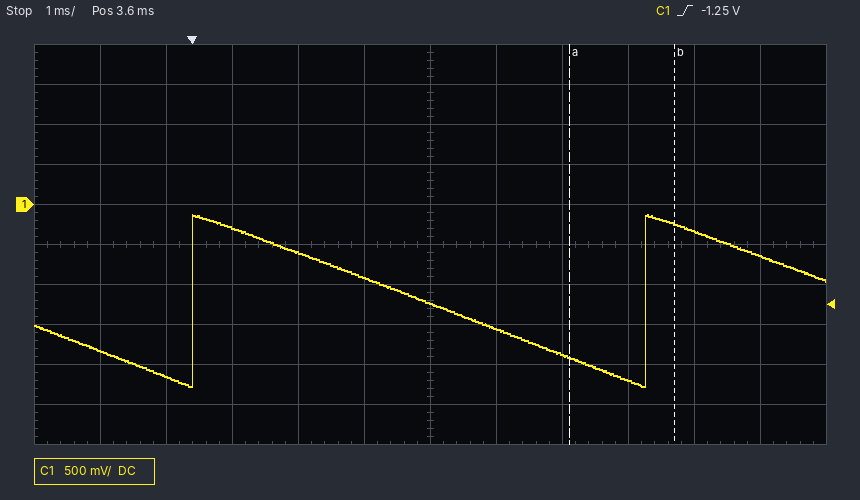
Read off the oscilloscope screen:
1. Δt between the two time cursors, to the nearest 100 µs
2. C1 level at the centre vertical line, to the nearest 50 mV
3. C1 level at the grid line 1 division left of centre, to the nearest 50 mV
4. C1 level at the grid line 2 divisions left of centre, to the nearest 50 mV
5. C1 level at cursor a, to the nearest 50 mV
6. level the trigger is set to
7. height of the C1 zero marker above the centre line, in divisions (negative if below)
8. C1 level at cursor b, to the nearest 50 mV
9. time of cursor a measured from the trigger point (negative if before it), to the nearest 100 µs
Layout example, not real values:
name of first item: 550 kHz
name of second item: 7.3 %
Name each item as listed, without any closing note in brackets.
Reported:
Δt between the two time cursors, to the nearest 100 µs: 1.6 ms
C1 level at the centre vertical line, to the nearest 50 mV: -1.25 V
C1 level at the grid line 1 division left of centre, to the nearest 50 mV: -900 mV
C1 level at the grid line 2 divisions left of centre, to the nearest 50 mV: -600 mV
C1 level at cursor a, to the nearest 50 mV: -1.90 V
level the trigger is set to: -1.25 V
height of the C1 zero marker above the centre line, in divisions: +1.0 div
C1 level at cursor b, to the nearest 50 mV: -250 mV
time of cursor a measured from the trigger point (negative if before it), to the nearest 100 µs: +5.7 ms
